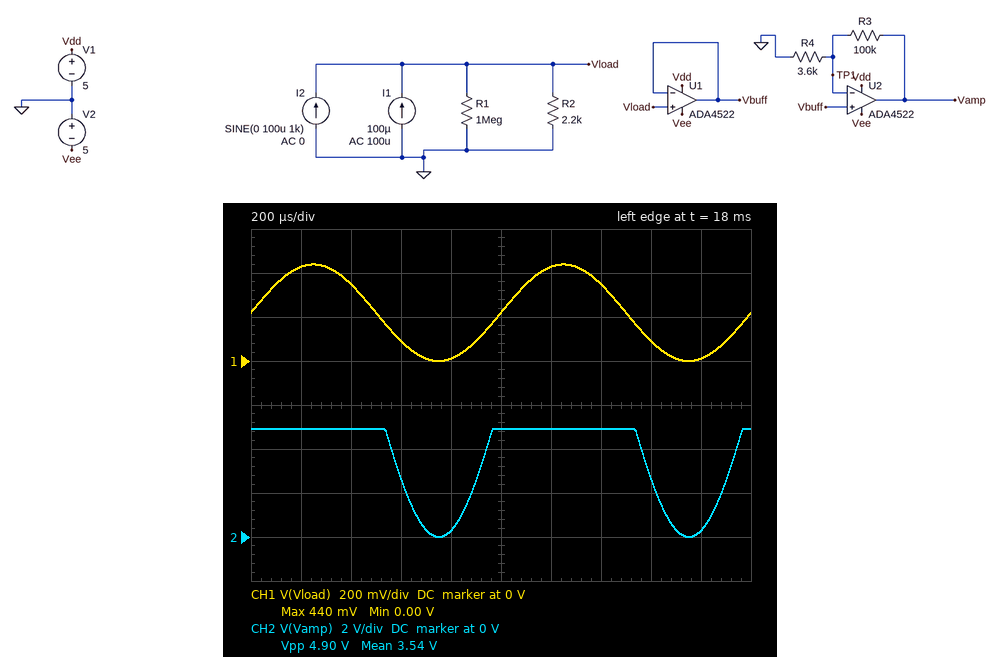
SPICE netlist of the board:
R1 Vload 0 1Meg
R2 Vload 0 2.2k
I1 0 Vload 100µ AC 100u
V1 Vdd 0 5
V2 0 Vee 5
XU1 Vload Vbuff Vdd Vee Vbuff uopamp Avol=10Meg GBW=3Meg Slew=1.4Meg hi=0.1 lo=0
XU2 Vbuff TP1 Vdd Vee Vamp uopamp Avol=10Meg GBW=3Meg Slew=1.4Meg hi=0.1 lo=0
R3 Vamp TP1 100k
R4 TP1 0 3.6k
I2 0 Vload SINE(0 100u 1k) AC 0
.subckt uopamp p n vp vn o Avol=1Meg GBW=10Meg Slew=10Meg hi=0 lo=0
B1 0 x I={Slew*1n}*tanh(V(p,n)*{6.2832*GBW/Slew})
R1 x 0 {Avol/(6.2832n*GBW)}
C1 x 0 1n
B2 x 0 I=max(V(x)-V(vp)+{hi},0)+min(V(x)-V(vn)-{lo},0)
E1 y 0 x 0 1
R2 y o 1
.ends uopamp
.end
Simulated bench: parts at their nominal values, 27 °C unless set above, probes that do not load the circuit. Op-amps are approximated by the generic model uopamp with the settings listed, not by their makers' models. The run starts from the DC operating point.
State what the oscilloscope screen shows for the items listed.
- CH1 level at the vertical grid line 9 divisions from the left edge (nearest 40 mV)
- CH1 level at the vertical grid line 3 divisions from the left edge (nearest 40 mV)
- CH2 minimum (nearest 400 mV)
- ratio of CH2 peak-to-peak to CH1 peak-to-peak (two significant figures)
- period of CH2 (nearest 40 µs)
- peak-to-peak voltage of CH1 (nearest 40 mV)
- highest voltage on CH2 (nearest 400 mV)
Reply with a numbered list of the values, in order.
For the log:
1. 0 V
2. 80 mV
3. 0 V
4. 11
5. 1.00 ms
6. 440 mV
7. 4.8 V
